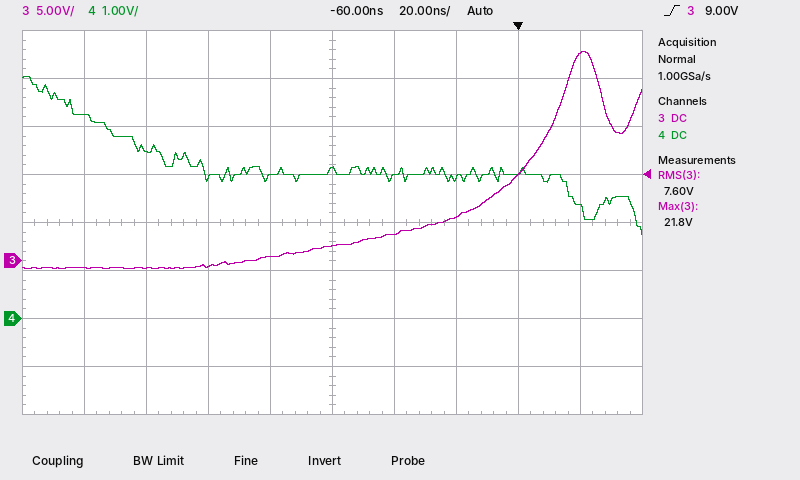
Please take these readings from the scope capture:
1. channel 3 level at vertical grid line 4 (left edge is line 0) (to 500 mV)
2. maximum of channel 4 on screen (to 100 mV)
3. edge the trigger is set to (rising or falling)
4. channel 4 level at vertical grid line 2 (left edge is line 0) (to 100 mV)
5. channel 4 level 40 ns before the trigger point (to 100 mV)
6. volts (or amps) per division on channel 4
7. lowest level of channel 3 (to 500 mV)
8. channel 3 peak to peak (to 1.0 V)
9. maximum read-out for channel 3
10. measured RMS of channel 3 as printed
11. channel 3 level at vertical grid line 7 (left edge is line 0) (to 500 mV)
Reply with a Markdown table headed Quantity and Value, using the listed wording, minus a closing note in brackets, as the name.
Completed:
| Quantity | Value |
|---|---|
| channel 3 level at vertical grid line 4 (left edge is line 0) | 500 mV |
| maximum of channel 4 on screen | 5.0 V |
| edge the trigger is set to | rising |
| channel 4 level at vertical grid line 2 (left edge is line 0) | 3.5 V |
| channel 4 level 40 ns before the trigger point | 3.0 V |
| volts (or amps) per division on channel 4 | 1 V |
| lowest level of channel 3 | -1.0 V |
| channel 3 peak to peak | 23.0 V |
| maximum read-out for channel 3 | 21.8 V |
| measured RMS of channel 3 as printed | 7.60 V |
| channel 3 level at vertical grid line 7 (left edge is line 0) | 4.5 V |
